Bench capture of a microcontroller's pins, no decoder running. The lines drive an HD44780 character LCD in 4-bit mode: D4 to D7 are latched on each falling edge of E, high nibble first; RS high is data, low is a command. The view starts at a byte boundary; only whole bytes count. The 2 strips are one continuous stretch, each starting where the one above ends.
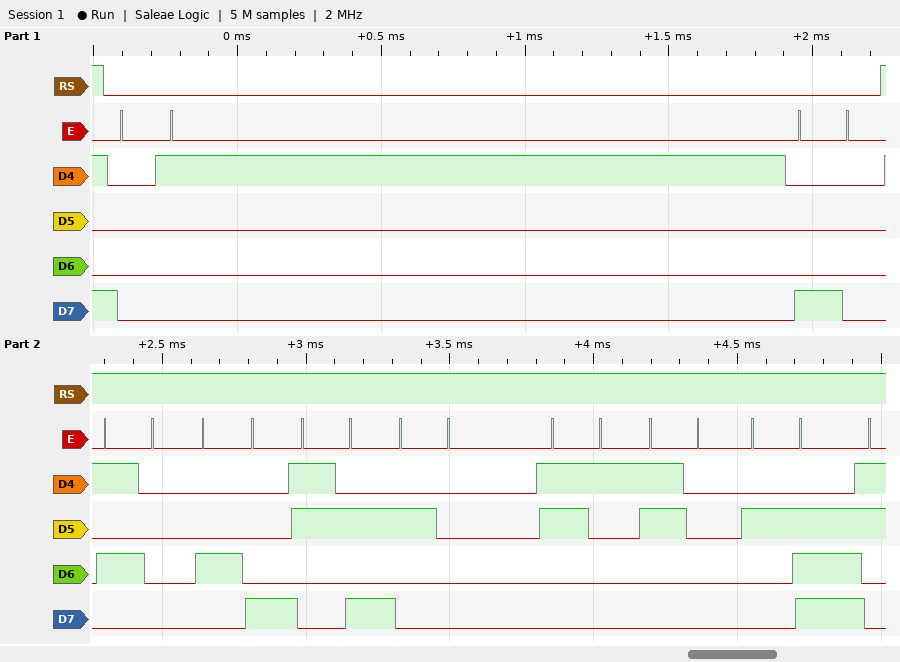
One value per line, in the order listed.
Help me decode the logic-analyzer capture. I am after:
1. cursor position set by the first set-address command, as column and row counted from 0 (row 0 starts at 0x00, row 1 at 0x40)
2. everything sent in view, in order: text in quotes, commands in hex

column 0, row 0
0x01 0x80 "PH: 10."
